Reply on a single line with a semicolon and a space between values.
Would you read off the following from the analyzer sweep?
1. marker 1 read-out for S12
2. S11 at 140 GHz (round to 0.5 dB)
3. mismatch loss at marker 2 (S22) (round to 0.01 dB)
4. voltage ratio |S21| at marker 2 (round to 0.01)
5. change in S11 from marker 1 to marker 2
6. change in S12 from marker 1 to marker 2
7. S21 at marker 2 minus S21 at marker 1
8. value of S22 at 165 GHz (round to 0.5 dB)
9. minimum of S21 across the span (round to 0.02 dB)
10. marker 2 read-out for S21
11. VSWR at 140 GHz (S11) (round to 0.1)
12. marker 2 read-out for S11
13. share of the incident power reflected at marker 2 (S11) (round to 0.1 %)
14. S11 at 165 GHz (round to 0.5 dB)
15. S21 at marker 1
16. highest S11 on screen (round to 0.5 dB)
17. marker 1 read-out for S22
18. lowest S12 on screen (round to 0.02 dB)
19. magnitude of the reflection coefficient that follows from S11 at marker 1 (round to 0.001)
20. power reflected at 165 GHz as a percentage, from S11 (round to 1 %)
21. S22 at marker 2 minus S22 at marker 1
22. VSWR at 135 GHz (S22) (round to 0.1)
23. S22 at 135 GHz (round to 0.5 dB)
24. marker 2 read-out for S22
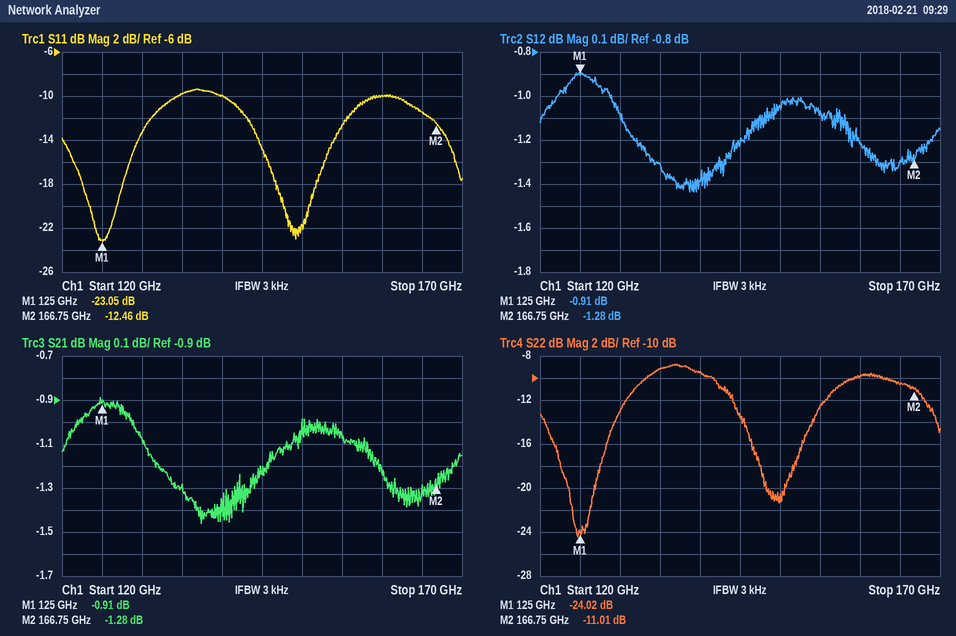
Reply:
-0.91 dB; -10.0 dB; 0.36 dB; 0.86; 10.59 dB; -0.37 dB; -0.37 dB; -10.5 dB; -1.46 dB; -1.28 dB; 1.9; -12.46 dB; 5.7 %; -11.5 dB; -0.91 dB; -9.5 dB; -24.02 dB; -1.44 dB; 0.070; 7 %; 13.01 dB; 2.1; -9.0 dB; -11.01 dB
